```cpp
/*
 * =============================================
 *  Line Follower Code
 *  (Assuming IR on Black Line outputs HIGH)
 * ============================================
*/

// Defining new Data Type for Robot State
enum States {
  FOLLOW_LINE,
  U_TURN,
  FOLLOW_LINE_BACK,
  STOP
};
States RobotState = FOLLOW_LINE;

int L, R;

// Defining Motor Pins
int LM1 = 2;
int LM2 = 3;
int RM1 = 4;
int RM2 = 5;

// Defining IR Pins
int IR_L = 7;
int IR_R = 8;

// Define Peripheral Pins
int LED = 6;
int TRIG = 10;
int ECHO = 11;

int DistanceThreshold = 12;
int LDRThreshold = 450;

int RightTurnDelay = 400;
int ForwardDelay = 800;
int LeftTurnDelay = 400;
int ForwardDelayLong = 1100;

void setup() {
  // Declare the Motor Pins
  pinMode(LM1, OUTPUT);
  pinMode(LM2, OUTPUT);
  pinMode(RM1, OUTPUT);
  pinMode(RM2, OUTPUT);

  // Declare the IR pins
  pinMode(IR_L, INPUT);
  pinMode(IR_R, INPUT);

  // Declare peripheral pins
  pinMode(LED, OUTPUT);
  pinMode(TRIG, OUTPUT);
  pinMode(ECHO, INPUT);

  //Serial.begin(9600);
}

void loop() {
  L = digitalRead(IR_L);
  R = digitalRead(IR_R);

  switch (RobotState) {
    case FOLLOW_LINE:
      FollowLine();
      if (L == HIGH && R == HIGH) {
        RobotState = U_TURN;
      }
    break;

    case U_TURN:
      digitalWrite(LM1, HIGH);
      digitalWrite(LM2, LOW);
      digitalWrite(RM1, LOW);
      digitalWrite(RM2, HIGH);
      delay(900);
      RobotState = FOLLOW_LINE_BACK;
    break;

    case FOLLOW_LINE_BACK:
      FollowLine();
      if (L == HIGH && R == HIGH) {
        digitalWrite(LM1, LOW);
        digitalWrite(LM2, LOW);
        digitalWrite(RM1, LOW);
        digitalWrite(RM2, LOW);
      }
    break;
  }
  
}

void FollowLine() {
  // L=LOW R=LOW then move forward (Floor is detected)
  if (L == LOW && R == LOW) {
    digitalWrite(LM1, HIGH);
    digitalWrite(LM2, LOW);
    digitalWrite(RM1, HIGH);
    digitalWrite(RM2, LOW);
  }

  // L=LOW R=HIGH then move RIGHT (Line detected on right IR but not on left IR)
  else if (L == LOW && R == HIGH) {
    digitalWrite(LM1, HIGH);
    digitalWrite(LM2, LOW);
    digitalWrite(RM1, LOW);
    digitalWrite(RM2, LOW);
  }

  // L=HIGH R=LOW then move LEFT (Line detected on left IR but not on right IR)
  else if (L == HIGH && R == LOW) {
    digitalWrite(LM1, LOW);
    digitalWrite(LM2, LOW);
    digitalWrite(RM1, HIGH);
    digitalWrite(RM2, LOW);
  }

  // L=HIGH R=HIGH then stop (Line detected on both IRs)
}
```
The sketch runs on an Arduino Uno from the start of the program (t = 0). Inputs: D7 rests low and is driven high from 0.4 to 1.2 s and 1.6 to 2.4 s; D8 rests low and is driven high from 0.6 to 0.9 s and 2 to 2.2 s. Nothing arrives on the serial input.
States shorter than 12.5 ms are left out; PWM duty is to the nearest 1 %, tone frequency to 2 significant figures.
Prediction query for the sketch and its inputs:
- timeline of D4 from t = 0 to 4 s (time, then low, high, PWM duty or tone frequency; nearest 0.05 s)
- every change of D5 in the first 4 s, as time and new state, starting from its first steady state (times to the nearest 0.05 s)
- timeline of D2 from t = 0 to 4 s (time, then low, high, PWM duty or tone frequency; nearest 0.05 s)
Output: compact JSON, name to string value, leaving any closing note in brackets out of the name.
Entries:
{"timeline of D4 from t = 0 to 4 s": "0 s high; 0.6 s low; 1.5 s high; 2 s low; 2.2 s high", "every change of D5 in the first 4 s, as time and new state, starting from its first steady state": "0 s low; 0.6 s high; 1.5 s low", "timeline of D2 from t = 0 to 4 s": "0 s high; 0.4 s low; 0.6 s high; 1.6 s low; 2.4 s high"}
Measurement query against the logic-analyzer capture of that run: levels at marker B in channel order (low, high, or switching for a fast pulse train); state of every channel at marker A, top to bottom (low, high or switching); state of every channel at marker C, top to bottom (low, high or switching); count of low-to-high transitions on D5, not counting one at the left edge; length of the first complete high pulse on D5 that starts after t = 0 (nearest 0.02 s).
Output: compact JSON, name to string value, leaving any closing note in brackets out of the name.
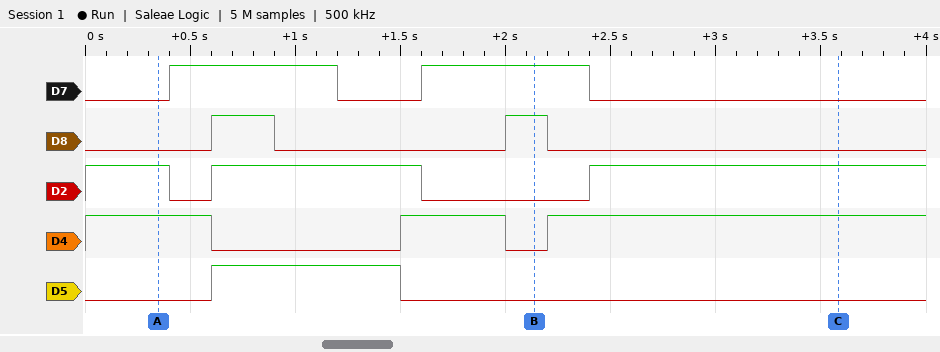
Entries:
{"levels at marker B in channel order": "D7 high, D8 high, D2 low, D4 low, D5 low", "state of every channel at marker A, top to bottom": "D7 low, D8 low, D2 high, D4 high, D5 low", "state of every channel at marker C, top to bottom": "D7 low, D8 low, D2 high, D4 high, D5 low", "count of low-to-high transitions on D5, not counting one at the left edge": "1", "length of the first complete high pulse on D5 that starts after t = 0": "0.90 s"}
